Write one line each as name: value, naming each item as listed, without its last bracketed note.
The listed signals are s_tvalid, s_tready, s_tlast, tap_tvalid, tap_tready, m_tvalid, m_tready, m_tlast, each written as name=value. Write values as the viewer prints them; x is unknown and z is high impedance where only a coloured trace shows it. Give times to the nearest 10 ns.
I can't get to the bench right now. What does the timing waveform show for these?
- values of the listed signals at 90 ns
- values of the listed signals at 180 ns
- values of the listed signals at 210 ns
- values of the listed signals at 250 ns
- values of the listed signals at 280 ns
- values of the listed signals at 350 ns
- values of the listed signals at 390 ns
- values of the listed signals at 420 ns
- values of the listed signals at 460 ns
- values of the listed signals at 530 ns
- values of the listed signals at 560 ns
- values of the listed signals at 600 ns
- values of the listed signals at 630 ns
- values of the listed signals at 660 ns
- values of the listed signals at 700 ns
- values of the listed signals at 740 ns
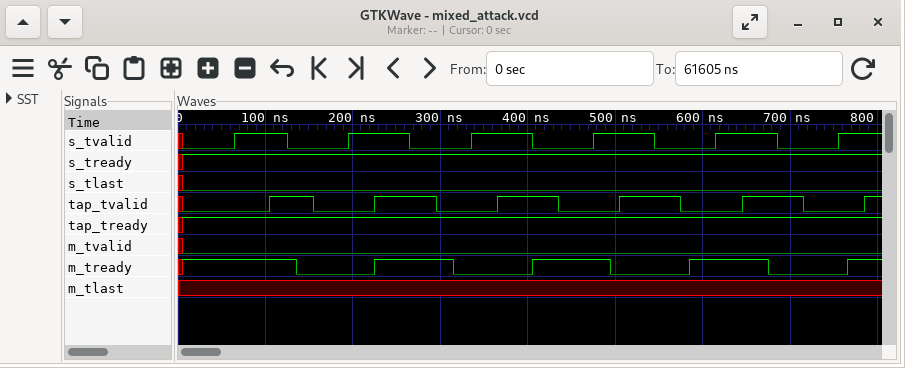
values of the listed signals at 90 ns: s_tvalid=1, s_tready=1, s_tlast=0, tap_tvalid=0, tap_tready=1, m_tvalid=0, m_tready=1, m_tlast=x
values of the listed signals at 180 ns: s_tvalid=0, s_tready=1, s_tlast=0, tap_tvalid=0, tap_tready=1, m_tvalid=0, m_tready=0, m_tlast=x
values of the listed signals at 210 ns: s_tvalid=1, s_tready=1, s_tlast=0, tap_tvalid=0, tap_tready=1, m_tvalid=0, m_tready=0, m_tlast=x
values of the listed signals at 250 ns: s_tvalid=1, s_tready=1, s_tlast=0, tap_tvalid=1, tap_tready=1, m_tvalid=0, m_tready=1, m_tlast=x
values of the listed signals at 280 ns: s_tvalid=0, s_tready=1, s_tlast=0, tap_tvalid=1, tap_tready=1, m_tvalid=0, m_tready=1, m_tlast=x
values of the listed signals at 350 ns: s_tvalid=1, s_tready=1, s_tlast=0, tap_tvalid=0, tap_tready=1, m_tvalid=0, m_tready=0, m_tlast=x
values of the listed signals at 390 ns: s_tvalid=1, s_tready=1, s_tlast=0, tap_tvalid=1, tap_tready=1, m_tvalid=0, m_tready=0, m_tlast=x
values of the listed signals at 420 ns: s_tvalid=0, s_tready=1, s_tlast=0, tap_tvalid=1, tap_tready=1, m_tvalid=0, m_tready=1, m_tlast=x
values of the listed signals at 460 ns: s_tvalid=0, s_tready=1, s_tlast=0, tap_tvalid=0, tap_tready=1, m_tvalid=0, m_tready=1, m_tlast=x
values of the listed signals at 530 ns: s_tvalid=1, s_tready=1, s_tlast=0, tap_tvalid=1, tap_tready=1, m_tvalid=0, m_tready=0, m_tlast=x
values of the listed signals at 560 ns: s_tvalid=0, s_tready=1, s_tlast=0, tap_tvalid=1, tap_tready=1, m_tvalid=0, m_tready=0, m_tlast=x
values of the listed signals at 600 ns: s_tvalid=0, s_tready=1, s_tlast=0, tap_tvalid=0, tap_tready=1, m_tvalid=0, m_tready=1, m_tlast=x
values of the listed signals at 630 ns: s_tvalid=1, s_tready=1, s_tlast=0, tap_tvalid=0, tap_tready=1, m_tvalid=0, m_tready=1, m_tlast=x
values of the listed signals at 660 ns: s_tvalid=1, s_tready=1, s_tlast=0, tap_tvalid=1, tap_tready=1, m_tvalid=0, m_tready=1, m_tlast=x
values of the listed signals at 700 ns: s_tvalid=0, s_tready=1, s_tlast=0, tap_tvalid=1, tap_tready=1, m_tvalid=0, m_tready=0, m_tlast=x
values of the listed signals at 740 ns: s_tvalid=0, s_tready=1, s_tlast=0, tap_tvalid=0, tap_tready=1, m_tvalid=0, m_tready=0, m_tlast=x
